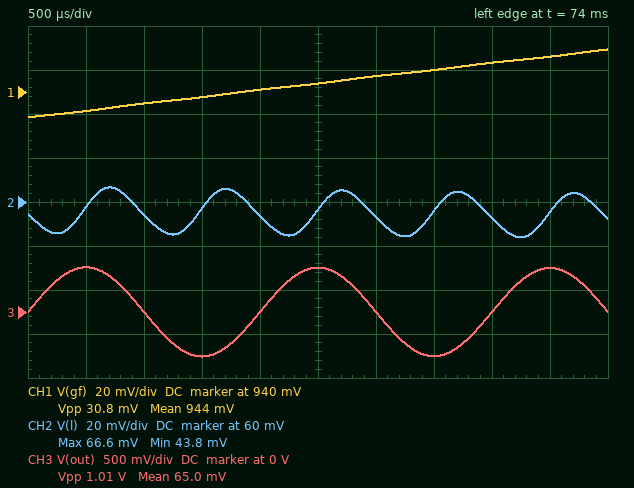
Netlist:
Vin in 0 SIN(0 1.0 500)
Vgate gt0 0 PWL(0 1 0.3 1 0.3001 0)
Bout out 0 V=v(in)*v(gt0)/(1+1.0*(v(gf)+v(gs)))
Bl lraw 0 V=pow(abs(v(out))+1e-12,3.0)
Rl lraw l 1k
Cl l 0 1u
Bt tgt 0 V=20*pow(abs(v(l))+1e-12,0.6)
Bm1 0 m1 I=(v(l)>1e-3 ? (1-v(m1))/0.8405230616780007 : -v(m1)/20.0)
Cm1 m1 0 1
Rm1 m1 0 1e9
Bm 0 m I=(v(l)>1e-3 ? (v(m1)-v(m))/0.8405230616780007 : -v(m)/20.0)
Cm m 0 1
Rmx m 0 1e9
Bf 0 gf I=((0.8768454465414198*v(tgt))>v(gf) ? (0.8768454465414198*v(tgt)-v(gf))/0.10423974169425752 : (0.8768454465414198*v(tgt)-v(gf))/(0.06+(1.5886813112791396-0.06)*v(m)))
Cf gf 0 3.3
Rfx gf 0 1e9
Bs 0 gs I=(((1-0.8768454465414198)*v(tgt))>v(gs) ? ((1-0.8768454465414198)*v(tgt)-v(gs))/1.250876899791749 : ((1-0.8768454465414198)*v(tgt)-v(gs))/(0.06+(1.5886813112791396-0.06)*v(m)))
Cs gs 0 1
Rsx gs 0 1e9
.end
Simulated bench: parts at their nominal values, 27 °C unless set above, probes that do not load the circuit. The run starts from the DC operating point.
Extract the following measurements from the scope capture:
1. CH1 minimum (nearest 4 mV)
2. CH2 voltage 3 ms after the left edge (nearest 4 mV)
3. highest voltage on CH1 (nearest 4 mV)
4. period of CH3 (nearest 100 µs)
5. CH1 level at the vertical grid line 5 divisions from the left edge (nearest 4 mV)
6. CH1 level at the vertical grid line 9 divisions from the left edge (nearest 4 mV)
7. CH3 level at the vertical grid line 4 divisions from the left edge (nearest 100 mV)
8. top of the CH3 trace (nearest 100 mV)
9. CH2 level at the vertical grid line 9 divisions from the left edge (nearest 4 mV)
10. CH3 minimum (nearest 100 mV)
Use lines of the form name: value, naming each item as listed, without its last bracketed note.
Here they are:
CH1 minimum: 928 mV
CH2 voltage 3 ms after the left edge: 52 mV
highest voltage on CH1: 960 mV
period of CH3: 2.0 ms
CH1 level at the vertical grid line 5 divisions from the left edge: 944 mV
CH1 level at the vertical grid line 9 divisions from the left edge: 956 mV
CH3 level at the vertical grid line 4 divisions from the left edge: 0 V
top of the CH3 trace: 500 mV
CH2 level at the vertical grid line 9 divisions from the left edge: 56 mV
CH3 minimum: -500 mV
